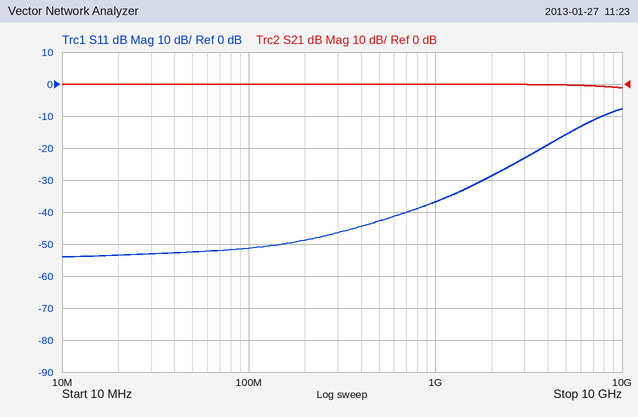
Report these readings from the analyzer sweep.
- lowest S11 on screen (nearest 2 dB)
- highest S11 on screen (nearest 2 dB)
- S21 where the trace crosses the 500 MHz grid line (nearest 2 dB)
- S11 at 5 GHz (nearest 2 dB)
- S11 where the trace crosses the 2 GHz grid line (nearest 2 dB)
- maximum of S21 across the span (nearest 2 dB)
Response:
-54 dB
-8 dB
0 dB
-16 dB
-28 dB
0 dB
